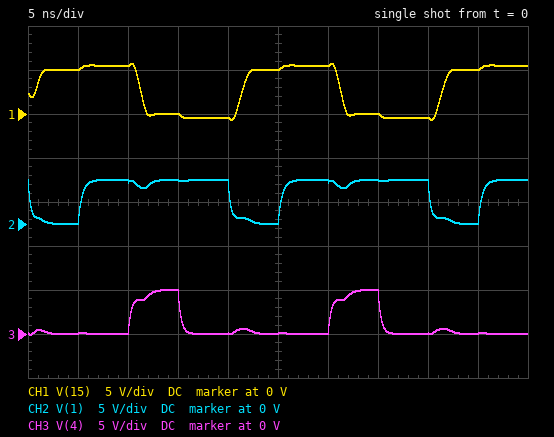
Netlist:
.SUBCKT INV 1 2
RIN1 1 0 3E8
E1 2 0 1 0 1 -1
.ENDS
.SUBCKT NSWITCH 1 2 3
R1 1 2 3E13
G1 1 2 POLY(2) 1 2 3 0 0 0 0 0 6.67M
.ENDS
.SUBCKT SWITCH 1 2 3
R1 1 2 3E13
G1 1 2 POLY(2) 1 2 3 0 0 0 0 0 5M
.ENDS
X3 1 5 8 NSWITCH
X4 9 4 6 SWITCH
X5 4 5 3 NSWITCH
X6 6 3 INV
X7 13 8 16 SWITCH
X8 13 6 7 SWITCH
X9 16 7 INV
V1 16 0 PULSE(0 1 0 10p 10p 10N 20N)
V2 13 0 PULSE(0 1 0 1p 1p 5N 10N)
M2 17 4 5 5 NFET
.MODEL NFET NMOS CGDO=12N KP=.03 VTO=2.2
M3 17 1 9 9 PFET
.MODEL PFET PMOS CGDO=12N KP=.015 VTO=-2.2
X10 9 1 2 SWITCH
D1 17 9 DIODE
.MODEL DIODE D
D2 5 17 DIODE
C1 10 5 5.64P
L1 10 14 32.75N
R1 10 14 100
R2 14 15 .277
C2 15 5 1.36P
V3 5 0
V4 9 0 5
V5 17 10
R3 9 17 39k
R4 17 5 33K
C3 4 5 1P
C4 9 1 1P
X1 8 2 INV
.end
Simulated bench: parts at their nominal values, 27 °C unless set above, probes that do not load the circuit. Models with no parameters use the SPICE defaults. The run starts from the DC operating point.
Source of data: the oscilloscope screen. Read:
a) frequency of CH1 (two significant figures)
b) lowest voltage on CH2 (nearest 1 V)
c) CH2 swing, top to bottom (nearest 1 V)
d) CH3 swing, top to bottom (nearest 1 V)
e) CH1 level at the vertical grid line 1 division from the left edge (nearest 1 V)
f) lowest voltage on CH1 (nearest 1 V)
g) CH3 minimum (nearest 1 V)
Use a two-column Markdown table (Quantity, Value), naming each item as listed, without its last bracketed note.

| Quantity | Value |
|---|---|
| frequency of CH1 | 50 MHz |
| lowest voltage on CH2 | 0 V |
| CH2 swing, top to bottom | 5 V |
| CH3 swing, top to bottom | 5 V |
| CH1 level at the vertical grid line 1 division from the left edge | 5 V |
| lowest voltage on CH1 | -1 V |
| CH3 minimum | 0 V |
